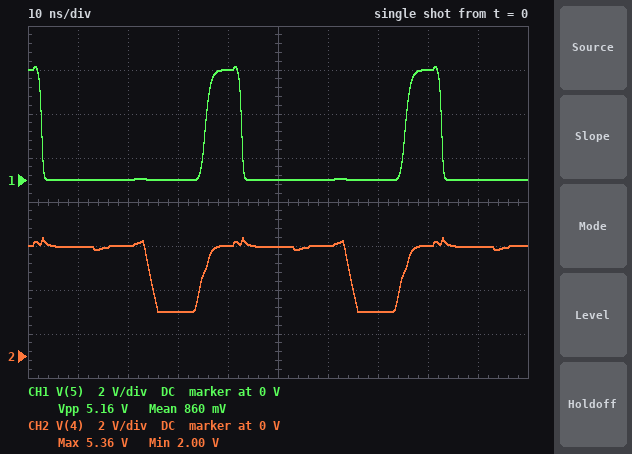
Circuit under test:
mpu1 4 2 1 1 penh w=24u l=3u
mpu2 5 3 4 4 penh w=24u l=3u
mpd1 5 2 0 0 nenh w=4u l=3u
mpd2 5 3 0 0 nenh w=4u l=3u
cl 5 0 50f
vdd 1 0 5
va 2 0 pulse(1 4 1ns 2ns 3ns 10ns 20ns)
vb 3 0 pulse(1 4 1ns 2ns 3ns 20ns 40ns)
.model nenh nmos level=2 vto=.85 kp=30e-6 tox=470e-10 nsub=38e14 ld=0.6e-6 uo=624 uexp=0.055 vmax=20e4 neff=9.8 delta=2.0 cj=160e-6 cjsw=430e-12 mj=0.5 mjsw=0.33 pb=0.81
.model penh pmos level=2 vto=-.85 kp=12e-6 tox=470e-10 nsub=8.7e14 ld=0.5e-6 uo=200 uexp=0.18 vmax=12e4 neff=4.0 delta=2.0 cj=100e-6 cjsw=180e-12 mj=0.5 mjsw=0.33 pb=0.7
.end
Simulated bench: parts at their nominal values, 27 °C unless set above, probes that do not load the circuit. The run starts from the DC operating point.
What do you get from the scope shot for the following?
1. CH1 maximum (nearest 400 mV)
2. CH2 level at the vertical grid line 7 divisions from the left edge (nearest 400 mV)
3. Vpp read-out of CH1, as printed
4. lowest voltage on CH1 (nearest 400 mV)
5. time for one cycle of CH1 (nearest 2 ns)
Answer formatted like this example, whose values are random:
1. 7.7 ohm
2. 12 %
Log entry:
1. 5.2 V
2. 2.0 V
3. 5.16 V
4. 0 V
5. 40 ns
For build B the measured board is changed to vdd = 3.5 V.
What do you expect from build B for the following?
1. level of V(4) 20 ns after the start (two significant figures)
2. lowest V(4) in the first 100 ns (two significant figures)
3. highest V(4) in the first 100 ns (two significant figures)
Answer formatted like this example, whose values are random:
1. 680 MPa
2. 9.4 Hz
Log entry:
1. 3.5 V
2. 1.0 V
3. 4.1 V
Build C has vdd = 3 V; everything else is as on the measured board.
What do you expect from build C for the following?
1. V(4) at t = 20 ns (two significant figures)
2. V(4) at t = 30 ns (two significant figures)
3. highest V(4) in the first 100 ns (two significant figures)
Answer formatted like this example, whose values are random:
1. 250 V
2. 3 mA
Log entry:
1. 3.0 V
2. 480 mV
3. 3.6 V
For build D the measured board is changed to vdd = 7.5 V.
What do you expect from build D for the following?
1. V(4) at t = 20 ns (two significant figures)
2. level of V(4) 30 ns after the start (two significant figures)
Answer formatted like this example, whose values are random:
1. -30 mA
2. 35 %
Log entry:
1. 7.0 V
2. 5.5 V
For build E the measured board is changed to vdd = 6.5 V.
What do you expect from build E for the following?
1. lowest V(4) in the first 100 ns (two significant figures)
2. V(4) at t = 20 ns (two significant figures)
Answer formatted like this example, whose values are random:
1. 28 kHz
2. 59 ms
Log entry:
1. 3.5 V
2. 6.2 V
